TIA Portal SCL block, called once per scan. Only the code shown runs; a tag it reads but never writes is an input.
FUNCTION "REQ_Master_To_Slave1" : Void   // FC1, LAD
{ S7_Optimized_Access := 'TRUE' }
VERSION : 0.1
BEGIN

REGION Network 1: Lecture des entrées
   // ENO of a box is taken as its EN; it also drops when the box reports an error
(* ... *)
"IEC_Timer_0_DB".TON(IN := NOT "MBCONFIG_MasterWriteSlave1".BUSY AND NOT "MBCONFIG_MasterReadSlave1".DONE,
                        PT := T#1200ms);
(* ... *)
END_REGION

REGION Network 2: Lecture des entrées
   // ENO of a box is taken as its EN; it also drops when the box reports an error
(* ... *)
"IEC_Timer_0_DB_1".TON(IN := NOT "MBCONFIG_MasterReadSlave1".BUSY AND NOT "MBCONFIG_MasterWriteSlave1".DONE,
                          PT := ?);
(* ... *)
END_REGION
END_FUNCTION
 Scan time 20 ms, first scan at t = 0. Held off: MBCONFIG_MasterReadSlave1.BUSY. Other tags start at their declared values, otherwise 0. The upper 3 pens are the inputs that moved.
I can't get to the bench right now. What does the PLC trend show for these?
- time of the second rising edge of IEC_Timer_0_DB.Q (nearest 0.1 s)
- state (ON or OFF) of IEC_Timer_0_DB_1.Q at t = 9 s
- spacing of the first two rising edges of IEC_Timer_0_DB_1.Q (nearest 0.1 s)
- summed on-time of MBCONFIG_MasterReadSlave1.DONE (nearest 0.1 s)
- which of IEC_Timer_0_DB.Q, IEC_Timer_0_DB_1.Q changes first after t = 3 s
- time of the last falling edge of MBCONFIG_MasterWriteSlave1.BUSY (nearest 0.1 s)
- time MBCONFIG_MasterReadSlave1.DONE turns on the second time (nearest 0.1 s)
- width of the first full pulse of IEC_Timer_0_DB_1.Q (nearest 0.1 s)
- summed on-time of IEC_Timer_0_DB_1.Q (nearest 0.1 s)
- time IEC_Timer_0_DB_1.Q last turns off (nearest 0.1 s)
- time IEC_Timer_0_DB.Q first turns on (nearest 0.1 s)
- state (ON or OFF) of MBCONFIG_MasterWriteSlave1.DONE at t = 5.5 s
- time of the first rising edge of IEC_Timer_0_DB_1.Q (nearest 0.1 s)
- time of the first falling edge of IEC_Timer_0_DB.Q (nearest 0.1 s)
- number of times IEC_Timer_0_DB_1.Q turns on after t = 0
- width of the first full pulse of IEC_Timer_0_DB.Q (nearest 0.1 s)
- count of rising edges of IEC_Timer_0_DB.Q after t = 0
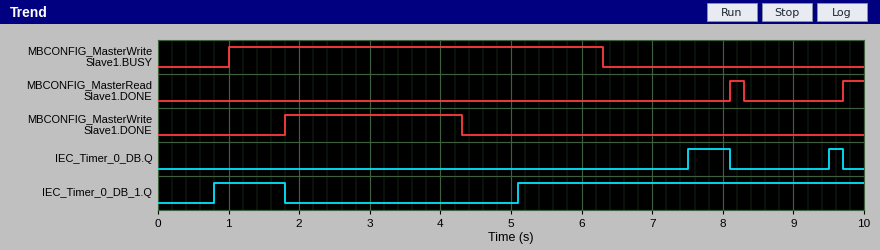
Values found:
9.5 s
ON
4.3 s
0.5 s
IEC_Timer_0_DB_1.Q
6.3 s
9.7 s
1.0 s
5.9 s
1.8 s
7.5 s
OFF
0.8 s
8.1 s
2
0.6 s
2
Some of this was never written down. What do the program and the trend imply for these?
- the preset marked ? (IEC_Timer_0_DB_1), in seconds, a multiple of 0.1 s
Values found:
0.8 s
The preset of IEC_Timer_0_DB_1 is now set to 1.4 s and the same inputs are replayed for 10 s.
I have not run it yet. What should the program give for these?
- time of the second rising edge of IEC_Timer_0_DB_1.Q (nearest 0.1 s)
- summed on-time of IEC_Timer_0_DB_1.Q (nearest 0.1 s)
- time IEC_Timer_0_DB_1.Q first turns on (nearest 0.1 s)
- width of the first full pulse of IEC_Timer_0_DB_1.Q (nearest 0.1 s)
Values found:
5.7 s
4.7 s
1.4 s
0.4 s
